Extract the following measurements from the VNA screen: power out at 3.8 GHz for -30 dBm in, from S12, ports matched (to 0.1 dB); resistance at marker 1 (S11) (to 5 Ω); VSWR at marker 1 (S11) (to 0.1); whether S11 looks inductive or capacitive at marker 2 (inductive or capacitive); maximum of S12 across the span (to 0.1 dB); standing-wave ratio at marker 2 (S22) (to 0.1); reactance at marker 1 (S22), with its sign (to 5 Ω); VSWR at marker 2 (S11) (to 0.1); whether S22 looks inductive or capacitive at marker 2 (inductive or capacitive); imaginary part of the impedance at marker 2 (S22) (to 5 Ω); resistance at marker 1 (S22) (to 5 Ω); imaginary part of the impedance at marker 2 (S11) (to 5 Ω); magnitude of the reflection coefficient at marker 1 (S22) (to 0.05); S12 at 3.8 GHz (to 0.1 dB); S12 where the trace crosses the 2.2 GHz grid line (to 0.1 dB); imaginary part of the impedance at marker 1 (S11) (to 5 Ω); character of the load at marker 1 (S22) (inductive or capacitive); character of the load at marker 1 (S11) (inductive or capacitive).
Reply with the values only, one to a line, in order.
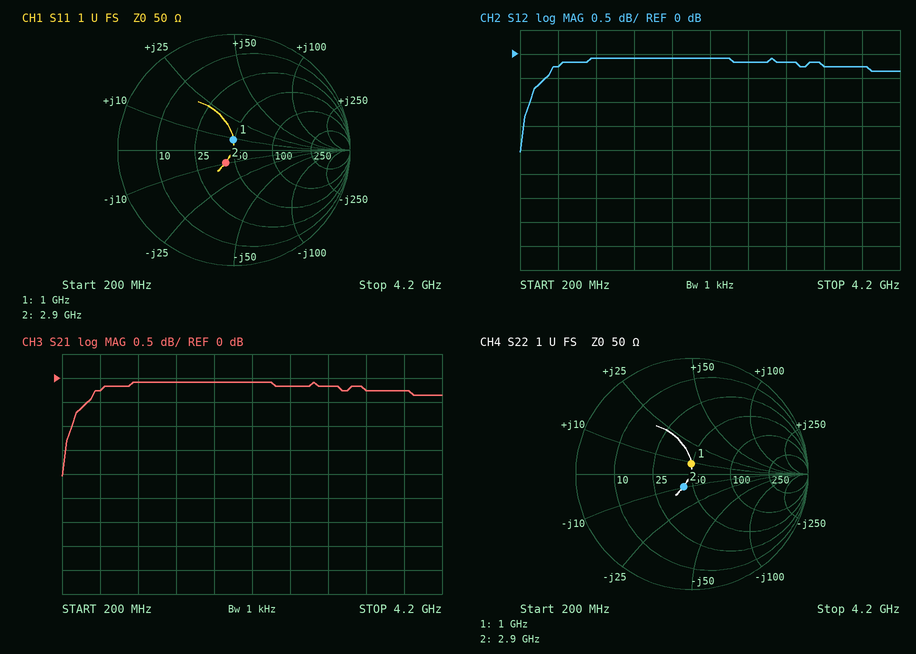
-30.3 dBm
50 Ω
1.2
capacitive
-0.1 dB
1.3
+10 Ω
1.3
capacitive
-10 Ω
50 Ω
-10 Ω
0.10
-0.3 dB
-0.1 dB
+10 Ω
inductive
inductive
